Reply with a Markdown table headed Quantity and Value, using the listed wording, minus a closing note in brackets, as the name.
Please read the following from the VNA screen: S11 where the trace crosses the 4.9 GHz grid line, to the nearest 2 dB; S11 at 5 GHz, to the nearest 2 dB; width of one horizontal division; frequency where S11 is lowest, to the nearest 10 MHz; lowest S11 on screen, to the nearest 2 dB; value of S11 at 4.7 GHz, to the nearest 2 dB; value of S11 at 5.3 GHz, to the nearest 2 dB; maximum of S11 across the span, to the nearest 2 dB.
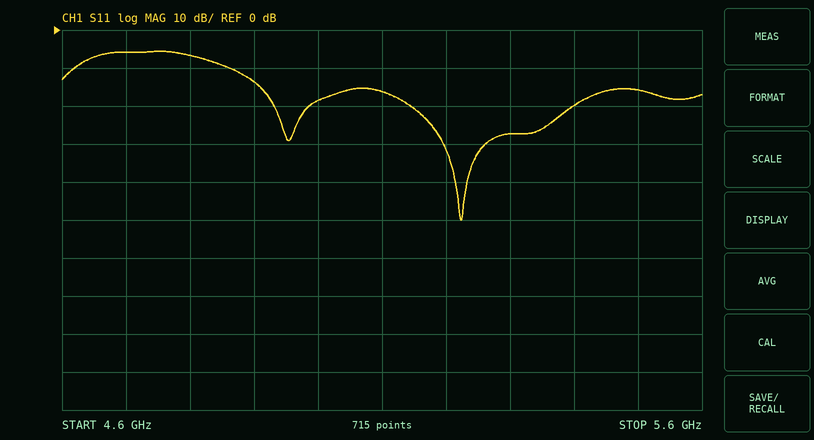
| Quantity | Value |
|---|---|
| S11 where the trace crosses the 4.9 GHz grid line, to the nearest 2 dB | -14 dB |
| S11 at 5 GHz, to the nearest 2 dB | -18 dB |
| width of one horizontal division | 100 MHz |
| frequency where S11 is lowest, to the nearest 10 MHz | 5.22 GHz |
| lowest S11 on screen, to the nearest 2 dB | -50 dB |
| value of S11 at 4.7 GHz, to the nearest 2 dB | -6 dB |
| value of S11 at 5.3 GHz, to the nearest 2 dB | -28 dB |
| maximum of S11 across the span, to the nearest 2 dB | -6 dB |
